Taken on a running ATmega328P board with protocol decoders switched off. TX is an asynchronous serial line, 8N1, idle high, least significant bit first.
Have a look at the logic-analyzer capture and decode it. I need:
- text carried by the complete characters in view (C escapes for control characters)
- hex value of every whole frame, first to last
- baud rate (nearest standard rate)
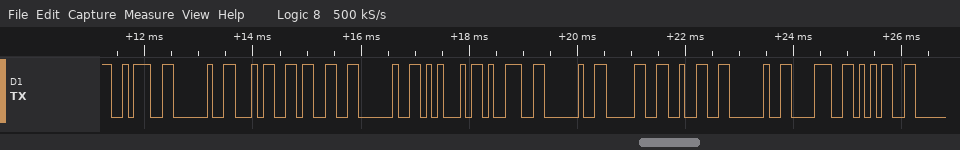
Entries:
": 43 E9 02 85"
3A 20 34 33 20 45 39 20 30 32 20 38 35
9600 baud
